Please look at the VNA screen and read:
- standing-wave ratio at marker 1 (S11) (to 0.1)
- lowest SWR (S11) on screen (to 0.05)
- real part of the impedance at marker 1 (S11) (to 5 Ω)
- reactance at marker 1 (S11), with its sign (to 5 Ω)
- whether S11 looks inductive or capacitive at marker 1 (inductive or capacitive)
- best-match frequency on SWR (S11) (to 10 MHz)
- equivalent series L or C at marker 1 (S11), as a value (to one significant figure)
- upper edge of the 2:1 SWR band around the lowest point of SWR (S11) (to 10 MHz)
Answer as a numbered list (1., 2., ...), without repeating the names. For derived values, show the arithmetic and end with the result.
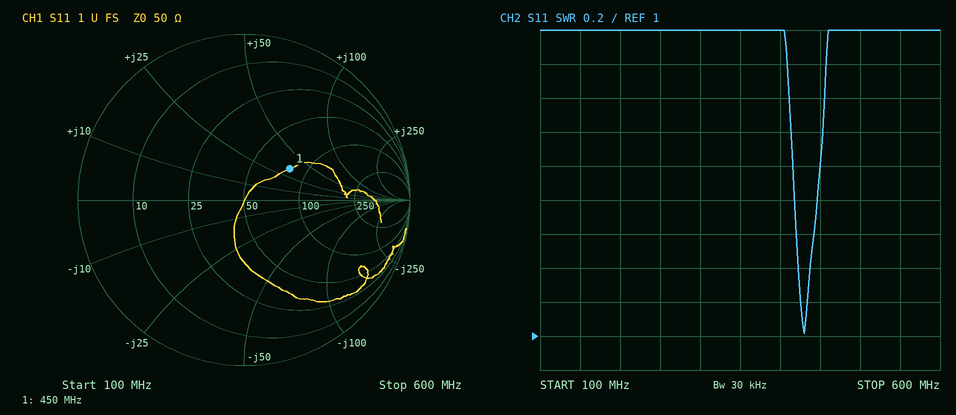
1. 2.0
2. 1.00
3. 80 Ω
4. +35 Ω
5. inductive
6. 430 MHz
7. L = 35 Ω/(2π × 450 MHz) ≈ 12.4 nH, so 10 nH to one significant figure
8. 450 MHz
